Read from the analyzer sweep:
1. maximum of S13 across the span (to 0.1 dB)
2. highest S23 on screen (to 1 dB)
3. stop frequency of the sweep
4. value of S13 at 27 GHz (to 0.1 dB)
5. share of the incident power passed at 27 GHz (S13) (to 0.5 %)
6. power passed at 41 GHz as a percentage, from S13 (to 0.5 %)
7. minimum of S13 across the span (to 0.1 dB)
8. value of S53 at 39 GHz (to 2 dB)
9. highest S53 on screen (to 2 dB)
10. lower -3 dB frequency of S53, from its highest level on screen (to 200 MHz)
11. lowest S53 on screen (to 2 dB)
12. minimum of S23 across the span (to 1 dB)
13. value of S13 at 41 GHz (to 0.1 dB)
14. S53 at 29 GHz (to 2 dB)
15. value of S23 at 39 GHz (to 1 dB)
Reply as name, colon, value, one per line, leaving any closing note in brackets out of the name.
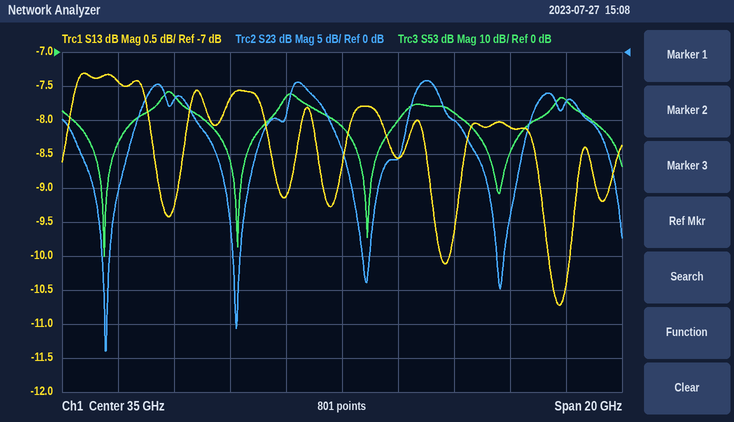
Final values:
maximum of S13 across the span: -7.3 dB
highest S23 on screen: -4 dB
stop frequency of the sweep: 45 GHz
value of S13 at 27 GHz: -7.4 dB
share of the incident power passed at 27 GHz (S13): 18.0 %
power passed at 41 GHz as a percentage, from S13: 15.5 %
minimum of S13 across the span: -10.7 dB
value of S53 at 39 GHz: -18 dB
highest S53 on screen: -12 dB
lower -3 dB frequency of S53, from its highest level on screen: 28.4 GHz
lowest S53 on screen: -60 dB
minimum of S23 across the span: -44 dB
value of S13 at 41 GHz: -8.1 dB
S53 at 29 GHz: -12 dB
value of S23 at 39 GHz: -10 dB
